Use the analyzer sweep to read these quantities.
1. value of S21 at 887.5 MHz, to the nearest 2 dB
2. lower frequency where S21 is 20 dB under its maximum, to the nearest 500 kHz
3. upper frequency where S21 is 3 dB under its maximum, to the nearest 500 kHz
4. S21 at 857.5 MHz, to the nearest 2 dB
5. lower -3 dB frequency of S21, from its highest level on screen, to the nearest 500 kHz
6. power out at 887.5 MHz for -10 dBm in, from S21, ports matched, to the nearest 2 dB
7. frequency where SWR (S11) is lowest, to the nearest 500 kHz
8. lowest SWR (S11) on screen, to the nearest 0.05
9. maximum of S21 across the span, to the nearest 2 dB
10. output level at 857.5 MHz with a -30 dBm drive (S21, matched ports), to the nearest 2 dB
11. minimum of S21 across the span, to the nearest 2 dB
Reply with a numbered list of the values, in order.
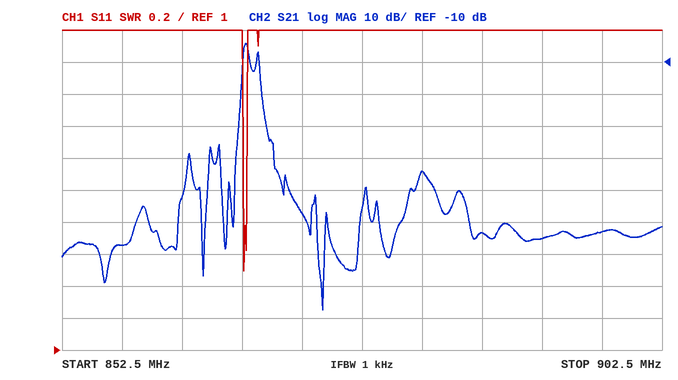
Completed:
1. -64 dB
2. 867.5 MHz
3. 868.0 MHz
4. -68 dB
5. 867.5 MHz
6. -74 dBm
7. 867.5 MHz
8. 1.50
9. -4 dB
10. -98 dBm
11. -88 dB
